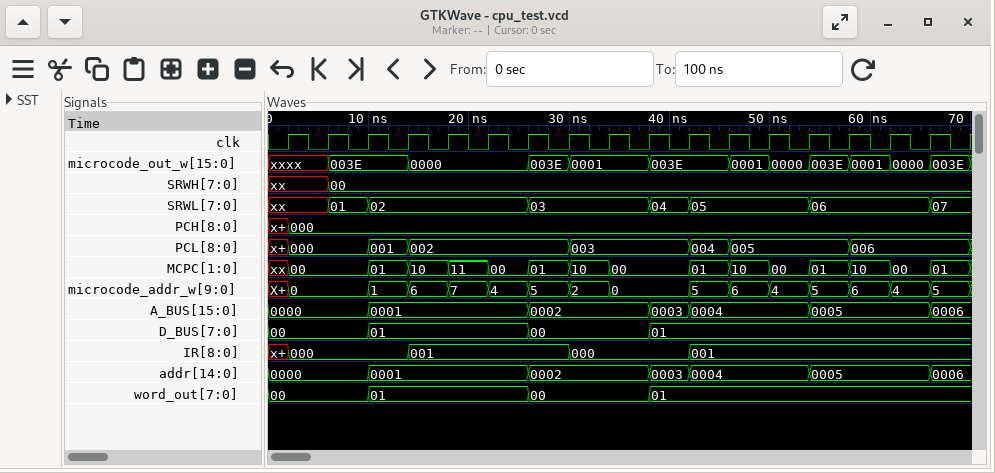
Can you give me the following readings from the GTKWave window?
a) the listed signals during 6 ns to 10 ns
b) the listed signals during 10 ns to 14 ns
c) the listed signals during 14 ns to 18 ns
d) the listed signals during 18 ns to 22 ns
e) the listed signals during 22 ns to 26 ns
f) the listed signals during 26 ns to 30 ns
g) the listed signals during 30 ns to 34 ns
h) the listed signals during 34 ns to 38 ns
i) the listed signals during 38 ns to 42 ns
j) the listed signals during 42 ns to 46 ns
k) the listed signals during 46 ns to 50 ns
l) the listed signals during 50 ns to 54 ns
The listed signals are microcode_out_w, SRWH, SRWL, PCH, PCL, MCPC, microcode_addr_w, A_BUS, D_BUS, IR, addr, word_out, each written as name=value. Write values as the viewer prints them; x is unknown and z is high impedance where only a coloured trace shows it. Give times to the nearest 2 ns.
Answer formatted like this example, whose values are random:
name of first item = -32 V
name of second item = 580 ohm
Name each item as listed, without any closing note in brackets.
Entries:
the listed signals during 6 ns to 10 ns = microcode_out_w=003E, SRWH=00, SRWL=01, PCH=000, PCL=000, MCPC=00, microcode_addr_w=0, A_BUS=0000, D_BUS=00, IR=000, addr=0000, word_out=00
the listed signals during 10 ns to 14 ns = microcode_out_w=003E, SRWH=00, SRWL=02, PCH=000, PCL=001, MCPC=01, microcode_addr_w=1, A_BUS=0001, D_BUS=01, IR=000, addr=0001, word_out=01
the listed signals during 14 ns to 18 ns = microcode_out_w=0000, SRWH=00, SRWL=02, PCH=000, PCL=002, MCPC=10, microcode_addr_w=6, A_BUS=0001, D_BUS=01, IR=001, addr=0001, word_out=01
the listed signals during 18 ns to 22 ns = microcode_out_w=0000, SRWH=00, SRWL=02, PCH=000, PCL=002, MCPC=11, microcode_addr_w=7, A_BUS=0001, D_BUS=01, IR=001, addr=0001, word_out=01
the listed signals during 22 ns to 26 ns = microcode_out_w=0000, SRWH=00, SRWL=02, PCH=000, PCL=002, MCPC=00, microcode_addr_w=4, A_BUS=0001, D_BUS=01, IR=001, addr=0001, word_out=01
the listed signals during 26 ns to 30 ns = microcode_out_w=003E, SRWH=00, SRWL=03, PCH=000, PCL=002, MCPC=01, microcode_addr_w=5, A_BUS=0002, D_BUS=00, IR=001, addr=0002, word_out=00
the listed signals during 30 ns to 34 ns = microcode_out_w=0001, SRWH=00, SRWL=03, PCH=000, PCL=003, MCPC=10, microcode_addr_w=2, A_BUS=0002, D_BUS=00, IR=000, addr=0002, word_out=00
the listed signals during 34 ns to 38 ns = microcode_out_w=0001, SRWH=00, SRWL=03, PCH=000, PCL=003, MCPC=00, microcode_addr_w=0, A_BUS=0002, D_BUS=00, IR=000, addr=0002, word_out=00
the listed signals during 38 ns to 42 ns = microcode_out_w=003E, SRWH=00, SRWL=04, PCH=000, PCL=003, MCPC=00, microcode_addr_w=0, A_BUS=0003, D_BUS=01, IR=000, addr=0003, word_out=01
the listed signals during 42 ns to 46 ns = microcode_out_w=003E, SRWH=00, SRWL=05, PCH=000, PCL=004, MCPC=01, microcode_addr_w=5, A_BUS=0004, D_BUS=01, IR=001, addr=0004, word_out=01
the listed signals during 46 ns to 50 ns = microcode_out_w=0001, SRWH=00, SRWL=05, PCH=000, PCL=005, MCPC=10, microcode_addr_w=6, A_BUS=0004, D_BUS=01, IR=001, addr=0004, word_out=01
the listed signals during 50 ns to 54 ns = microcode_out_w=0000, SRWH=00, SRWL=05, PCH=000, PCL=005, MCPC=00, microcode_addr_w=4, A_BUS=0004, D_BUS=01, IR=001, addr=0004, word_out=01
